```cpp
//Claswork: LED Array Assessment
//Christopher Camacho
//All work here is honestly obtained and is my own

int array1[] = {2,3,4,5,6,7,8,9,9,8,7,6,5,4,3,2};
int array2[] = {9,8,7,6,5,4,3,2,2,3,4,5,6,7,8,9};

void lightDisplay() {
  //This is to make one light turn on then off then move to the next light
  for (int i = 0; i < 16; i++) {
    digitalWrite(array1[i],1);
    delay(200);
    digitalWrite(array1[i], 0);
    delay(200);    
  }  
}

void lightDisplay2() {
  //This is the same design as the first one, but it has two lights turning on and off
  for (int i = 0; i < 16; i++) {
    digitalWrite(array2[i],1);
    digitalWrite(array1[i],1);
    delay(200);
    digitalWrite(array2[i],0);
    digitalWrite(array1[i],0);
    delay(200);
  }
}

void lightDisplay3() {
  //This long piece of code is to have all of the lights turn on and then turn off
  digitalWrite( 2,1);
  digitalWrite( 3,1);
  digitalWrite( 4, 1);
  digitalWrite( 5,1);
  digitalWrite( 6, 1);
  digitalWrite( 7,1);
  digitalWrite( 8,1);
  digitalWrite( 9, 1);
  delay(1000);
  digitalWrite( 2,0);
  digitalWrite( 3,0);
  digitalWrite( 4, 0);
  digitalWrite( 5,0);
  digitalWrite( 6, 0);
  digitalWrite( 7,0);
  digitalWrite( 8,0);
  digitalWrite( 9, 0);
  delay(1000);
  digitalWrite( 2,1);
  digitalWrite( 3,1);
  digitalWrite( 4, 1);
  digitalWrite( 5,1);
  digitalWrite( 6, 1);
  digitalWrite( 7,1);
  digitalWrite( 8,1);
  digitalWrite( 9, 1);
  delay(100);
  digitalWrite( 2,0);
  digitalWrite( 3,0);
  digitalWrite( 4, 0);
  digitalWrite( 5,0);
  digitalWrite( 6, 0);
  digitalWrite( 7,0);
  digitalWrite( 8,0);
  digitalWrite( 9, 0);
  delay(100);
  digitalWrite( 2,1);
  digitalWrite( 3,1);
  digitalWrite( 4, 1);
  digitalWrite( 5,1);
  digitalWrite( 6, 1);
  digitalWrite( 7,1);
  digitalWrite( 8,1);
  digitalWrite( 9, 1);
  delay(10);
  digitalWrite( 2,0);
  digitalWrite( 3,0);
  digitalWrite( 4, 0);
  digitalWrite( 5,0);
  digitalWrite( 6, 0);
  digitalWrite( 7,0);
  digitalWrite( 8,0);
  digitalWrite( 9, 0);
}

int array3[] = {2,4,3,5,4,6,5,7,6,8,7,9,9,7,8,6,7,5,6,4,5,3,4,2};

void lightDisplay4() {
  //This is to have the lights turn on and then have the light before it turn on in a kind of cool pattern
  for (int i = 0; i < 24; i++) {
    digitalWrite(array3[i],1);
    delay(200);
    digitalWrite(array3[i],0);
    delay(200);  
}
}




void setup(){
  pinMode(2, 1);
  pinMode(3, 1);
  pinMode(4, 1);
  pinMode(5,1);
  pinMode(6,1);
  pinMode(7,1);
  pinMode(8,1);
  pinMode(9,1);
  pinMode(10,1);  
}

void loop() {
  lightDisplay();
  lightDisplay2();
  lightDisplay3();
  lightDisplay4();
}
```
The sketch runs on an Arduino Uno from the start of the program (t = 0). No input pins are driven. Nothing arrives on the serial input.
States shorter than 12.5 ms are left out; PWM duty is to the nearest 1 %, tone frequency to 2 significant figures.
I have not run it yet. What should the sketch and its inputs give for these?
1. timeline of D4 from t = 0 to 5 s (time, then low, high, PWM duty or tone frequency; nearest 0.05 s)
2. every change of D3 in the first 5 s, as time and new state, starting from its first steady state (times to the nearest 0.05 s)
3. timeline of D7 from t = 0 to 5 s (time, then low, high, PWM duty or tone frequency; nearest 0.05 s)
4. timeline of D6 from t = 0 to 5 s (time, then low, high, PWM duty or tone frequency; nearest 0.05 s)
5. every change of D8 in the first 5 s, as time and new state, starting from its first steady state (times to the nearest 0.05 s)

0 s low; 0.8 s high; 1 s low
0 s low; 0.4 s high; 0.6 s low
0 s low; 2 s high; 2.2 s low; 4 s high; 4.2 s low
0 s low; 1.6 s high; 1.8 s low; 4.4 s high; 4.6 s low
0 s low; 2.4 s high; 2.6 s low; 3.6 s high; 3.8 s low
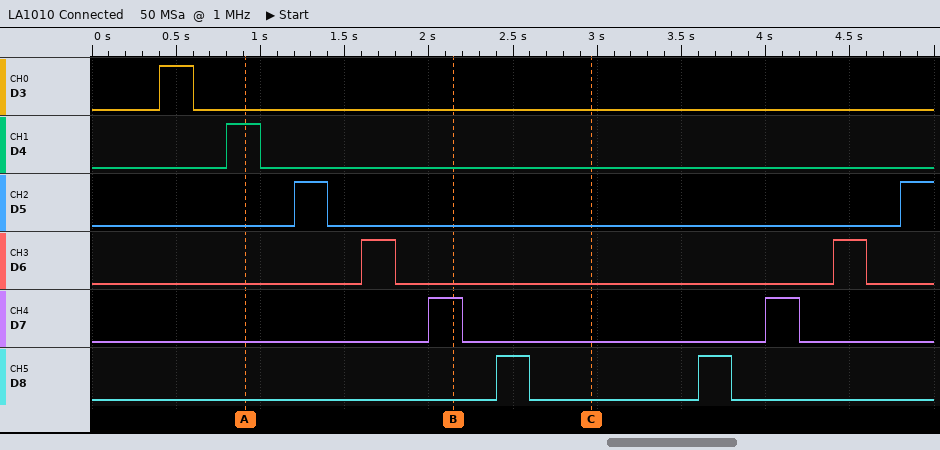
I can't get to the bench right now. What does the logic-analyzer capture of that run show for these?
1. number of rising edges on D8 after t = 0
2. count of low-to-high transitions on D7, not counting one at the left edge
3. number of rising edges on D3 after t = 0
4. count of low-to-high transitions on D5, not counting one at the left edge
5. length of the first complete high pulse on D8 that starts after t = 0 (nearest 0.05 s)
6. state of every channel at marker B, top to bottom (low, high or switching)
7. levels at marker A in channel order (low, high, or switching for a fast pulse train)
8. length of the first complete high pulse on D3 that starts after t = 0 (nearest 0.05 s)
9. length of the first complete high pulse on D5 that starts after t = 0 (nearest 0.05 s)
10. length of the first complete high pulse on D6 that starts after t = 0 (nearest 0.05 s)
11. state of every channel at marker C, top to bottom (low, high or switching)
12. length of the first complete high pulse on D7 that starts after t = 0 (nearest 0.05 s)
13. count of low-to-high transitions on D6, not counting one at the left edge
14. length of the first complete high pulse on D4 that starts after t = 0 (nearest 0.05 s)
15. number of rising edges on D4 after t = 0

2
2
1
2
0.20 s
D3 low, D4 low, D5 low, D6 low, D7 high, D8 low
D3 low, D4 high, D5 low, D6 low, D7 low, D8 low
0.20 s
0.20 s
0.20 s
D3 low, D4 low, D5 low, D6 low, D7 low, D8 low
0.20 s
2
0.20 s
1
